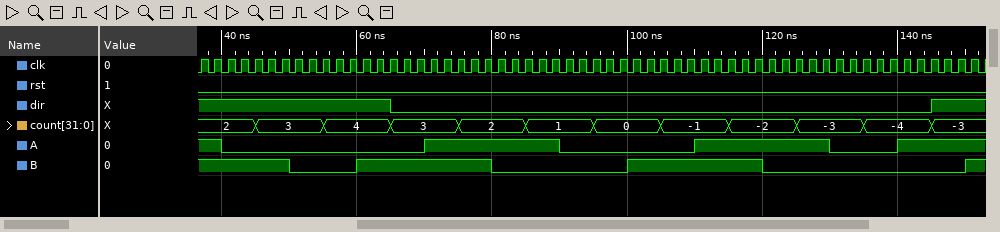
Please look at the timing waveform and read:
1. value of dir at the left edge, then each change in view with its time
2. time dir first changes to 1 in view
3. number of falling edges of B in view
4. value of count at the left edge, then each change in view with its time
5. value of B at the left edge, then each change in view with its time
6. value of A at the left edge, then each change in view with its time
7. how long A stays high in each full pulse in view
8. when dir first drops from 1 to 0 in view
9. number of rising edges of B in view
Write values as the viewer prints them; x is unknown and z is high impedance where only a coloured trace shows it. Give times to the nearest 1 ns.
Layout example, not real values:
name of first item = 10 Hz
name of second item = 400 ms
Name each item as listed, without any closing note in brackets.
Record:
value of dir at the left edge, then each change in view with its time = 1, 0 at 65 ns, 1 at 145 ns
time dir first changes to 1 in view = 145 ns
number of falling edges of B in view = 3
value of count at the left edge, then each change in view with its time = 2, 3 at 45 ns, 4 at 55 ns, 3 at 65 ns, 2 at 75 ns, 1 at 85 ns, 0 at 95 ns, -1 at 105 ns, -2 at 115 ns, -3 at 125 ns, -4 at 135 ns, -3 at 145 ns
value of B at the left edge, then each change in view with its time = 1, 0 at 50 ns, 1 at 60 ns, 0 at 80 ns, 1 at 100 ns, 0 at 120 ns, 1 at 150 ns
value of A at the left edge, then each change in view with its time = 1, 0 at 40 ns, 1 at 70 ns, 0 at 90 ns, 1 at 110 ns, 0 at 130 ns, 1 at 140 ns
how long A stays high in each full pulse in view = 20 ns, 20 ns
when dir first drops from 1 to 0 in view = 65 ns
number of rising edges of B in view = 3
